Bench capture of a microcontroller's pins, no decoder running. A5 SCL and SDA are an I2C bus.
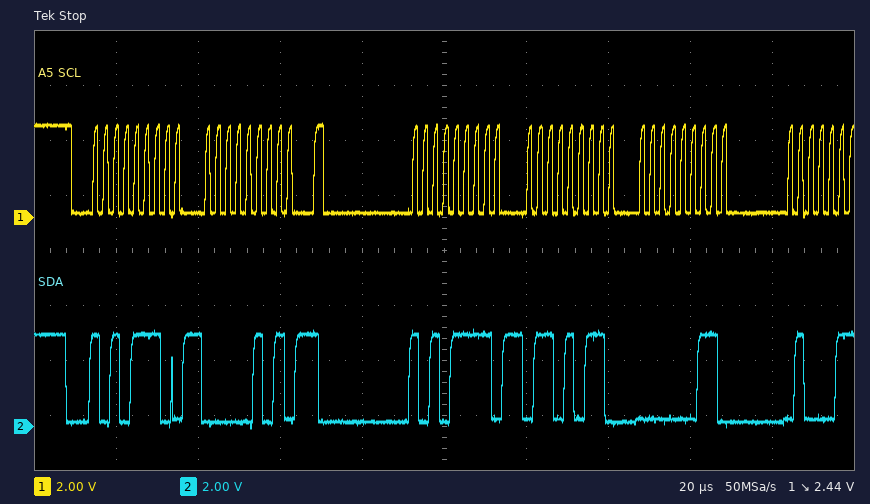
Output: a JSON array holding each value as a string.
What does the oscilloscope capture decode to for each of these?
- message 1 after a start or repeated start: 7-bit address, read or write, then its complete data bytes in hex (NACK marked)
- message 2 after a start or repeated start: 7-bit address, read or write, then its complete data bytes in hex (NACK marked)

["0x57 write: 05", "0x57 read: 6B 03"]
